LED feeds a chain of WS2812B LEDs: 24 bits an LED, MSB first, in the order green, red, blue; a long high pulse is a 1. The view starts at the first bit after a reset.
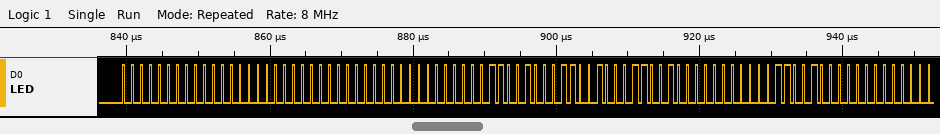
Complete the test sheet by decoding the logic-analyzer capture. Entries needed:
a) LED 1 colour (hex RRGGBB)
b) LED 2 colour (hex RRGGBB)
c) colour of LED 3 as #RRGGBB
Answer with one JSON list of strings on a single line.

["#000000", "#000064", "#646400"]
